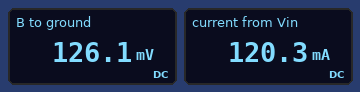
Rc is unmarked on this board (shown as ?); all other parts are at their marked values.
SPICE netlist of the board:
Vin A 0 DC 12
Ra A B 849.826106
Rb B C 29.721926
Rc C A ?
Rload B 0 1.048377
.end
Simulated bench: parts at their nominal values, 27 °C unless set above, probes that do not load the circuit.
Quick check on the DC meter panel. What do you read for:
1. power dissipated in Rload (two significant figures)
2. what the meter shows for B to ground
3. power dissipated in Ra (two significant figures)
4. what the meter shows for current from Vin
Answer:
15 mW
126.1 mV
170 mW
120.3 mA
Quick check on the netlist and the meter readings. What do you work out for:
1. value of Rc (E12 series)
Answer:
82 Ω
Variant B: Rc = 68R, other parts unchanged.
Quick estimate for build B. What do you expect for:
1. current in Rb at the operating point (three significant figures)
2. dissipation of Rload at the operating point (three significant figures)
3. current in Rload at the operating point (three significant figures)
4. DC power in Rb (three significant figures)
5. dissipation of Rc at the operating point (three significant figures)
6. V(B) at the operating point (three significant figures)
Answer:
121 mA
19.2 mW
135 mA
438 mW
1.00 W
142 mV
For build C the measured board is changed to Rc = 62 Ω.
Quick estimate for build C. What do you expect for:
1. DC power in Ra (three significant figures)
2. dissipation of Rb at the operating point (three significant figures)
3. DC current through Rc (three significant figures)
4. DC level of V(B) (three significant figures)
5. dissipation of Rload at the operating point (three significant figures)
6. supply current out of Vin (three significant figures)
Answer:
165 mW
496 mW
129 mA
150 mV
21.5 mW
143 mA
